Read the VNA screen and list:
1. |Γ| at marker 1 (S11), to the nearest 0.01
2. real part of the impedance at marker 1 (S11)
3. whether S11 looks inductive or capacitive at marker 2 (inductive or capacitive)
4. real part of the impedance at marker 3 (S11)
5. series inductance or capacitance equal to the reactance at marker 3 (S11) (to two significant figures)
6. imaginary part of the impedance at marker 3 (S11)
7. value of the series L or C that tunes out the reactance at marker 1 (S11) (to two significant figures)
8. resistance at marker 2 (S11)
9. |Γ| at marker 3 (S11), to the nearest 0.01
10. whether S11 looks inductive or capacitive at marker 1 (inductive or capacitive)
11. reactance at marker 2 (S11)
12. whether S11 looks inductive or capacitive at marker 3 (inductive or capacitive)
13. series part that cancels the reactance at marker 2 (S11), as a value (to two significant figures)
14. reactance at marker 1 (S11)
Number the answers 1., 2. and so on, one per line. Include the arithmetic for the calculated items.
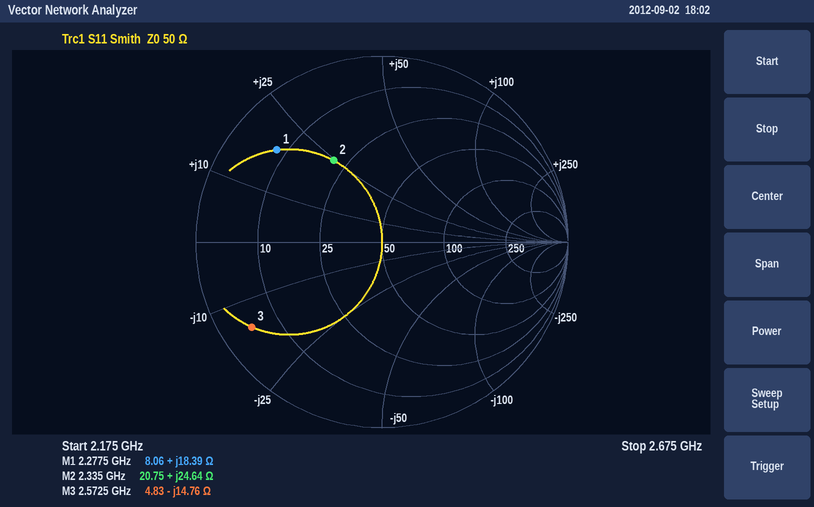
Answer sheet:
1. 0.75
2. 8.06 Ω
3. inductive
4. 4.83 Ω
5. C = 1/(2π × 2.5725 GHz × 14.76 Ω) ≈ 4.2 pF
6. -14.76 Ω
7. C = 1/(2π × 2.2775 GHz × 18.39 Ω) ≈ 3.8 pF
8. 20.75 Ω
9. 0.84
10. inductive
11. +24.64 Ω
12. capacitive
13. C = 1/(2π × 2.335 GHz × 24.64 Ω) ≈ 2.8 pF
14. +18.39 Ω
